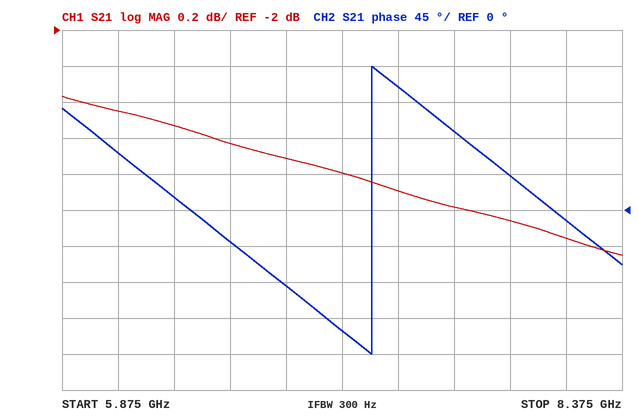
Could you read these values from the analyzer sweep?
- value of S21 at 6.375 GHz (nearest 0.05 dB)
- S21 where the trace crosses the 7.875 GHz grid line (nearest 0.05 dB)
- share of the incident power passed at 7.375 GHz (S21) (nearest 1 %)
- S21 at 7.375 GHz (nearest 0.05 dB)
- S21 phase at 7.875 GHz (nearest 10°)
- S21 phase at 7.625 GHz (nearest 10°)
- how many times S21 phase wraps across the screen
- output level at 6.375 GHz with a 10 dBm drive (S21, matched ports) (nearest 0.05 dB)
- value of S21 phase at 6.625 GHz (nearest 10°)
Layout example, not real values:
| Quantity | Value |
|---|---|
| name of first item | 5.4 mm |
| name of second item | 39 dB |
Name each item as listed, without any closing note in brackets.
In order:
| Quantity | Value |
|---|---|
| value of S21 at 6.375 GHz | -2.55 dB |
| S21 where the trace crosses the 7.875 GHz grid line | -3.05 dB |
| share of the incident power passed at 7.375 GHz (S21) | 51 % |
| S21 at 7.375 GHz | -2.90 dB |
| S21 phase at 7.875 GHz | 40° |
| S21 phase at 7.625 GHz | 100° |
| how many times S21 phase wraps across the screen | 1 |
| output level at 6.375 GHz with a 10 dBm drive (S21, matched ports) | 7.45 dBm |
| value of S21 phase at 6.625 GHz | -40° |
